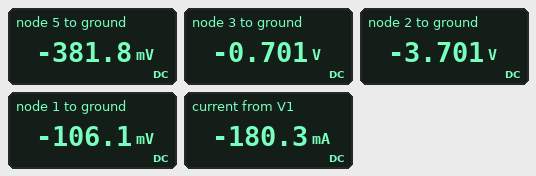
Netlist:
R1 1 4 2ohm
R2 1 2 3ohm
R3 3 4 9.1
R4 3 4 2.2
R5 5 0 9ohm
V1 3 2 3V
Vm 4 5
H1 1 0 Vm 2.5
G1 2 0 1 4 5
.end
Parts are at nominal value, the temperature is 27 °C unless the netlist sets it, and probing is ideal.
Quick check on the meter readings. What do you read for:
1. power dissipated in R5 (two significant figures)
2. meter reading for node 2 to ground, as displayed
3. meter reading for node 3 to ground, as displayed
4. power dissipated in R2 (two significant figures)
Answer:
16 mW
-3.701 V
-0.701 V
4.3 W
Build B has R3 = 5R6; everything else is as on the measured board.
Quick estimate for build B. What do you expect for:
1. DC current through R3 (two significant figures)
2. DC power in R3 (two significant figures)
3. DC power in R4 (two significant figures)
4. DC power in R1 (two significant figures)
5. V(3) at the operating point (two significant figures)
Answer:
50 mA
14 mW
36 mW
37 mW
-660 mV
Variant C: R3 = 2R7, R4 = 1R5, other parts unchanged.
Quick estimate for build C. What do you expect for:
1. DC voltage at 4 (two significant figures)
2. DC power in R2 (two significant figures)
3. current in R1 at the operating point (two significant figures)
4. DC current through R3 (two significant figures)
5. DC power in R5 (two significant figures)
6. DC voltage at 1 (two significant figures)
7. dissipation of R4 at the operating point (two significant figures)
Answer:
-360 mV
3.9 W
130 mA
61 mA
15 mW
-100 mV
18 mW
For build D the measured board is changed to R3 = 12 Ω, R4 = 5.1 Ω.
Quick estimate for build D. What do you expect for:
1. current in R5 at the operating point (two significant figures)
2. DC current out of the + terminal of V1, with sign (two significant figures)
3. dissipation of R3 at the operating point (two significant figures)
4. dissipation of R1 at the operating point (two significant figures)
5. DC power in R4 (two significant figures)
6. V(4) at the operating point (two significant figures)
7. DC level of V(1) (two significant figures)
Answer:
48 mA
-200 mA
44 mW
48 mW
100 mW
-430 mV
-120 mV
